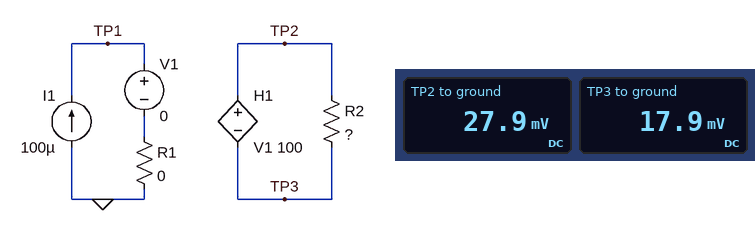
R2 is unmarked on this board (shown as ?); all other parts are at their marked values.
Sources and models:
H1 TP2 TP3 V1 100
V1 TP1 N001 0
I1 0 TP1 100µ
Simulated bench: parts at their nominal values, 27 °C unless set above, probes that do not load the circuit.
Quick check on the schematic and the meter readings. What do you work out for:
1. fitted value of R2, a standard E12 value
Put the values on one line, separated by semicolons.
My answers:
0.56 Ω
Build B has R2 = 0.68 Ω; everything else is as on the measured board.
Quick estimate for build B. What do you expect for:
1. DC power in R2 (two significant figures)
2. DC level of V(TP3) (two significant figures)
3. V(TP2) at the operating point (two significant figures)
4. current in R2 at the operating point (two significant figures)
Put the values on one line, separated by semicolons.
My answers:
150 µW; 15 mV; 25 mV; 15 mA
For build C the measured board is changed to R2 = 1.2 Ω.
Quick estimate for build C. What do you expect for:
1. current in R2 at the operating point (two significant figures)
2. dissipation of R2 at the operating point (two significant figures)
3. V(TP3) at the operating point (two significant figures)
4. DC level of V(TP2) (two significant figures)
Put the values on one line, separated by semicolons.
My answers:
8.3 mA; 83 µW; 8.3 mV; 18 mV
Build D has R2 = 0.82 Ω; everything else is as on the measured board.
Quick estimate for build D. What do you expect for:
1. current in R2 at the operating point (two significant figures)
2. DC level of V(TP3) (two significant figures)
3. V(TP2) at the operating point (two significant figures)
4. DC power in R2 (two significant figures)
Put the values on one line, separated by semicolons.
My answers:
12 mA; 12 mV; 22 mV; 120 µW
